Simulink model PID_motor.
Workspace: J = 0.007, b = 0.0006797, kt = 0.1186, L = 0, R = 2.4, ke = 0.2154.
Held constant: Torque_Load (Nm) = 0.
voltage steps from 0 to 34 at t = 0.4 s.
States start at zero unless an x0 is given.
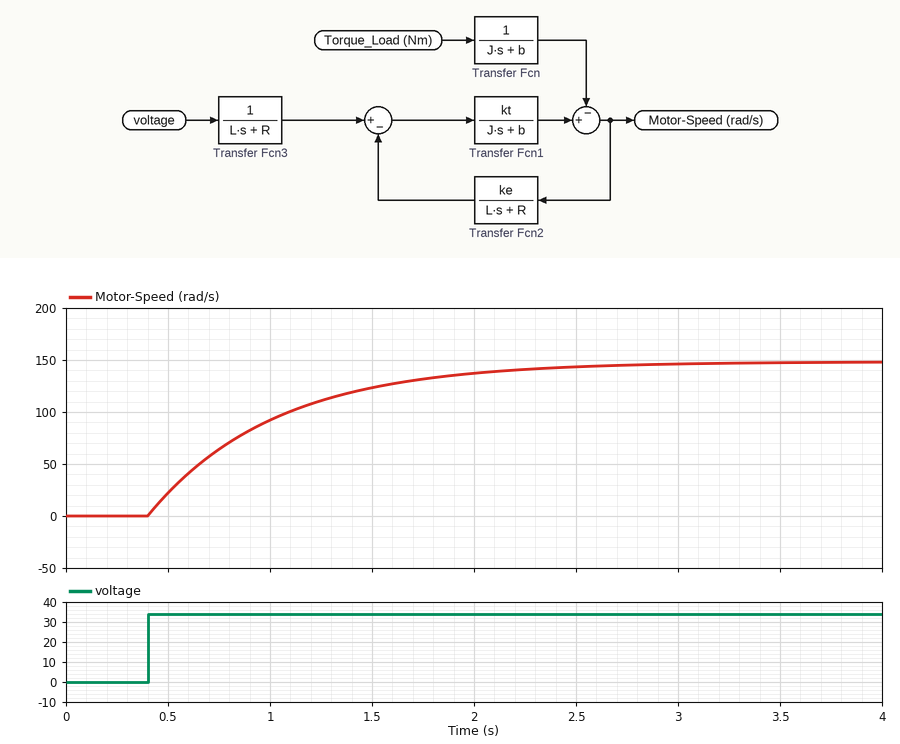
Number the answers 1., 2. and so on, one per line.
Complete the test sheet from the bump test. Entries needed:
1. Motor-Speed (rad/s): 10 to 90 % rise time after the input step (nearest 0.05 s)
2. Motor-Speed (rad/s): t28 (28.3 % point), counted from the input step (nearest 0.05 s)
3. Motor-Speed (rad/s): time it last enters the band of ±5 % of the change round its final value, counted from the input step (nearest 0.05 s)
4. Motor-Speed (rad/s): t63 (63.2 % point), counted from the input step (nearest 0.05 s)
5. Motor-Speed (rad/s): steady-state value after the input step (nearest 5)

1. 1.35 s
2. 0.20 s
3. 1.85 s
4. 0.60 s
5. 150
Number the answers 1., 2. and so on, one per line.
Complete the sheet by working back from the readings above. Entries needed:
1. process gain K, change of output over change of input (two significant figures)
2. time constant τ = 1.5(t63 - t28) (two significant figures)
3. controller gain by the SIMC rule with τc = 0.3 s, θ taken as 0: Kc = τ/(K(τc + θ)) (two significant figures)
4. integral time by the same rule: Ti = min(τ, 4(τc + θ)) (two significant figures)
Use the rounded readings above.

1. 4.4
2. 0.60 s
3. 0.45
4. 0.60 s
